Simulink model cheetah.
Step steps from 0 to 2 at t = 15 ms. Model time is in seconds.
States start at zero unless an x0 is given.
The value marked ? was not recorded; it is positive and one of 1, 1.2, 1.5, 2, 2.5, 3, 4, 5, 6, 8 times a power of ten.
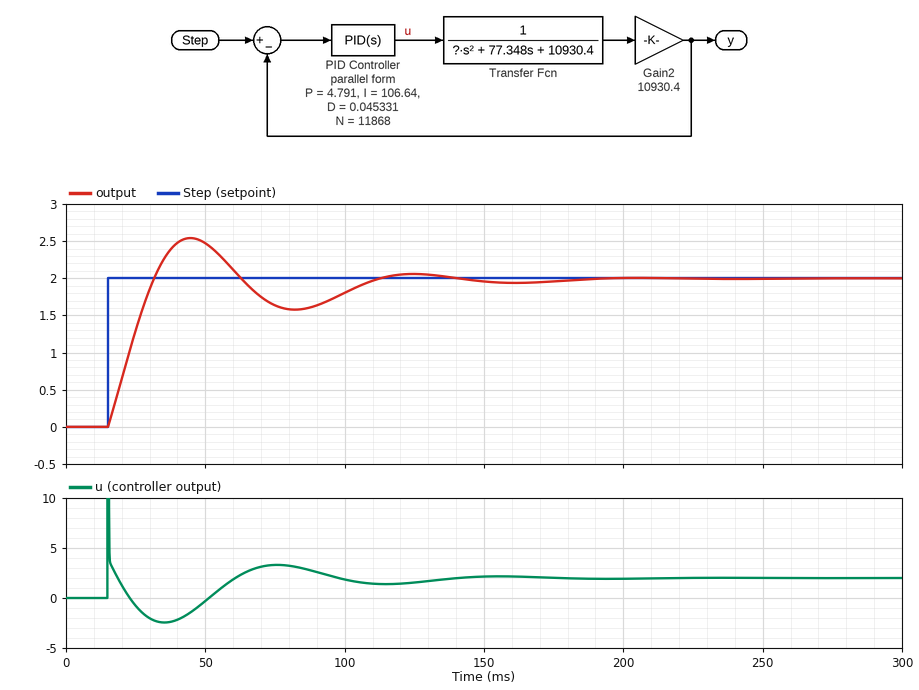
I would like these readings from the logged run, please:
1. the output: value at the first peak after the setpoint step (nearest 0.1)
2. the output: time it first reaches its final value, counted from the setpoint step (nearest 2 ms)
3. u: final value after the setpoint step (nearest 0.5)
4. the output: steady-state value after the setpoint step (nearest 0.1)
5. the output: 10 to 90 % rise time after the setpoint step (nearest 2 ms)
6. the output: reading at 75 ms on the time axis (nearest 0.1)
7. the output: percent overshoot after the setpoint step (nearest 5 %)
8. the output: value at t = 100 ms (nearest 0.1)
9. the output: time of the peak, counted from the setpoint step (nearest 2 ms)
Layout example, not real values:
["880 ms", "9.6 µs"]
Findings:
["2.5", "16 ms", "2.0", "2.0", "12 ms", "1.6", "25 %", "1.8", "30 ms"]
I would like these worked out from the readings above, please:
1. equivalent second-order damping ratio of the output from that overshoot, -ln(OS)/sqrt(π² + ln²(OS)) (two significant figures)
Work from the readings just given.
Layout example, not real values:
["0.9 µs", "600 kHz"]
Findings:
["0.40"]
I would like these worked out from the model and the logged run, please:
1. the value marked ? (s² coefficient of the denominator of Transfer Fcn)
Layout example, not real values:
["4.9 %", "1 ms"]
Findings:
["8"]
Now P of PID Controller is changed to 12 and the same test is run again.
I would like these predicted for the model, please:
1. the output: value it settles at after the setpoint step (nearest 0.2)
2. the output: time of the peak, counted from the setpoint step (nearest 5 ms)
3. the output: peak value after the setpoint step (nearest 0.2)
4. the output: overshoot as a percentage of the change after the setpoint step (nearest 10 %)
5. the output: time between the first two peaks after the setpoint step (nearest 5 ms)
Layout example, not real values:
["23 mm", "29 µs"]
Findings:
["2.0", "20 ms", "2.8", "40 %", "50 ms"]
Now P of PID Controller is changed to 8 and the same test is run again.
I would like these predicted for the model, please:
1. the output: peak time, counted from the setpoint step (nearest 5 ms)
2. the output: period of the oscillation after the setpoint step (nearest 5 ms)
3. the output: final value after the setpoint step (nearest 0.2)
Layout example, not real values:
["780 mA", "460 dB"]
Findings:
["25 ms", "60 ms", "2.0"]
